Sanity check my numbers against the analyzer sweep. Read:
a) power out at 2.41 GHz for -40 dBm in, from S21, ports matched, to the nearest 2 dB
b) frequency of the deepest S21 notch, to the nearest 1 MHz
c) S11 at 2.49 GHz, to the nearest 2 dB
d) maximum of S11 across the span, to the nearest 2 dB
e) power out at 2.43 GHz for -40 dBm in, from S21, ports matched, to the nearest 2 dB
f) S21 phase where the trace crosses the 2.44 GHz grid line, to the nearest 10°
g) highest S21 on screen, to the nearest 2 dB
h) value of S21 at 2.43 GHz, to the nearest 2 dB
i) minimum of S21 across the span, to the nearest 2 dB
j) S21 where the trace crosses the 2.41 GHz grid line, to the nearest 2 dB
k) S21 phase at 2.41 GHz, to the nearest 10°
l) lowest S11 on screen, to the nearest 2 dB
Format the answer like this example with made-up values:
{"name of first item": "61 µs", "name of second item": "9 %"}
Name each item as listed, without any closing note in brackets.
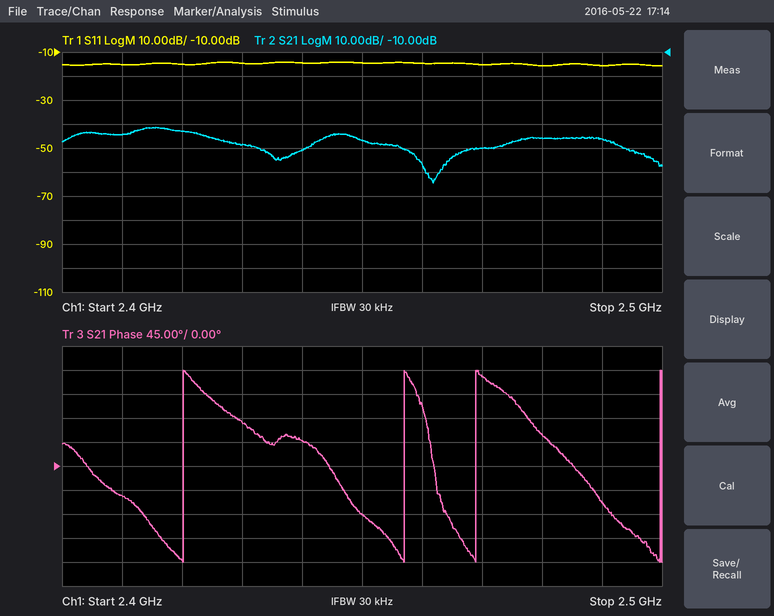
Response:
{"power out at 2.41 GHz for -40 dBm in, from S21, ports matched, to the nearest 2 dB": "-84 dBm", "frequency of the deepest S21 notch, to the nearest 1 MHz": "2.462 GHz", "S11 at 2.49 GHz, to the nearest 2 dB": "-16 dB", "maximum of S11 across the span, to the nearest 2 dB": "-14 dB", "power out at 2.43 GHz for -40 dBm in, from S21, ports matched, to the nearest 2 dB": "-88 dBm", "S21 phase where the trace crosses the 2.44 GHz grid line, to the nearest 10°": "50°", "highest S21 on screen, to the nearest 2 dB": "-42 dB", "value of S21 at 2.43 GHz, to the nearest 2 dB": "-48 dB", "minimum of S21 across the span, to the nearest 2 dB": "-64 dB", "S21 where the trace crosses the 2.41 GHz grid line, to the nearest 2 dB": "-44 dB", "S21 phase at 2.41 GHz, to the nearest 10°": "-60°", "lowest S11 on screen, to the nearest 2 dB": "-16 dB"}
